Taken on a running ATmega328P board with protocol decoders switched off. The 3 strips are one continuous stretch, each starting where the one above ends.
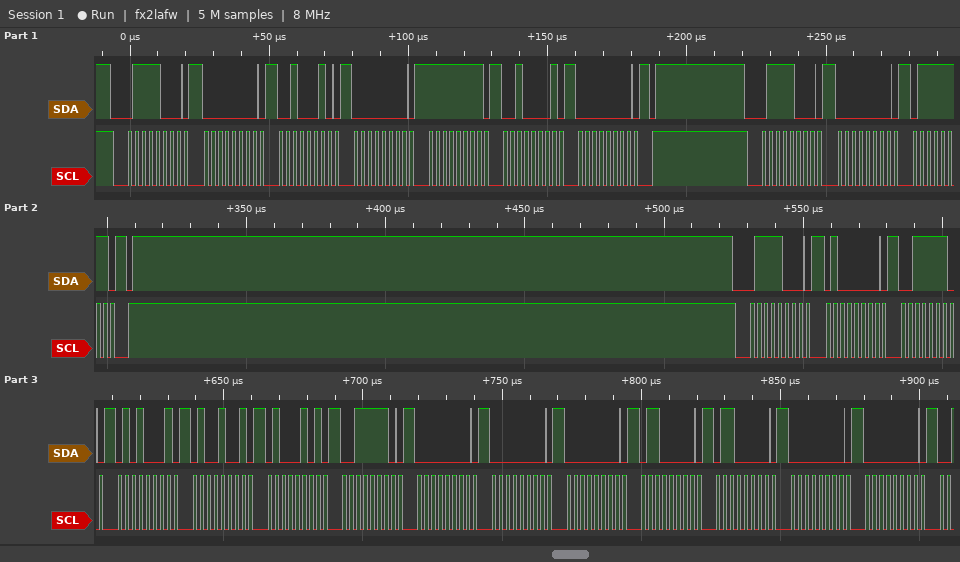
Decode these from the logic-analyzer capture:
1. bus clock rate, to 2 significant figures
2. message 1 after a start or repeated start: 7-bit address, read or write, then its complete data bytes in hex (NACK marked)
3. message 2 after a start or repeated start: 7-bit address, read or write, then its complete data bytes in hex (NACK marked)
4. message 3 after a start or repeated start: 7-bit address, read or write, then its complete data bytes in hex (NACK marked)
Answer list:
400 kHz
0x3C write: 00 22 00 FF 21 00
0x3C write: 00 7F
0x3C write: 40 3E 51 49 45 3E 00 00 00 60 60 00 00
